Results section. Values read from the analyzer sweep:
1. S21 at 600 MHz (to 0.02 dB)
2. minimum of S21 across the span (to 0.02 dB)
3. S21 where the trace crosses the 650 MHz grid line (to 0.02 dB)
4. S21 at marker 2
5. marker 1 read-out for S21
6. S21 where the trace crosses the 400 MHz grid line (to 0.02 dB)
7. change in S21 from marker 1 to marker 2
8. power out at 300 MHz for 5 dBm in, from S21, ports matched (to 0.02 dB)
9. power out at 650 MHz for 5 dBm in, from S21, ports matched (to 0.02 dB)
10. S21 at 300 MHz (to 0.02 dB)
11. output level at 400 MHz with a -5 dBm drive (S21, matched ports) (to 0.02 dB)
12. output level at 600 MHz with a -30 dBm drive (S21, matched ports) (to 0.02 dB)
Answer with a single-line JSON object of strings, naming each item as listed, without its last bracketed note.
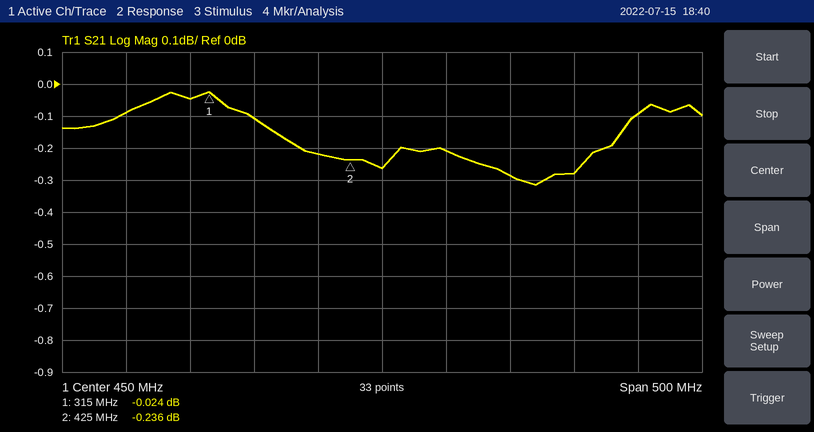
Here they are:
{"S21 at 600 MHz": "-0.28 dB", "minimum of S21 across the span": "-0.32 dB", "S21 where the trace crosses the 650 MHz grid line": "-0.10 dB", "S21 at marker 2": "-0.236 dB", "marker 1 read-out for S21": "-0.024 dB", "S21 where the trace crosses the 400 MHz grid line": "-0.22 dB", "change in S21 from marker 1 to marker 2": "-0.212 dB", "power out at 300 MHz for 5 dBm in, from S21, ports matched": "4.96 dBm", "power out at 650 MHz for 5 dBm in, from S21, ports matched": "4.90 dBm", "S21 at 300 MHz": "-0.04 dB", "output level at 400 MHz with a -5 dBm drive (S21, matched ports)": "-5.22 dBm", "output level at 600 MHz with a -30 dBm drive (S21, matched ports)": "-30.28 dBm"}
